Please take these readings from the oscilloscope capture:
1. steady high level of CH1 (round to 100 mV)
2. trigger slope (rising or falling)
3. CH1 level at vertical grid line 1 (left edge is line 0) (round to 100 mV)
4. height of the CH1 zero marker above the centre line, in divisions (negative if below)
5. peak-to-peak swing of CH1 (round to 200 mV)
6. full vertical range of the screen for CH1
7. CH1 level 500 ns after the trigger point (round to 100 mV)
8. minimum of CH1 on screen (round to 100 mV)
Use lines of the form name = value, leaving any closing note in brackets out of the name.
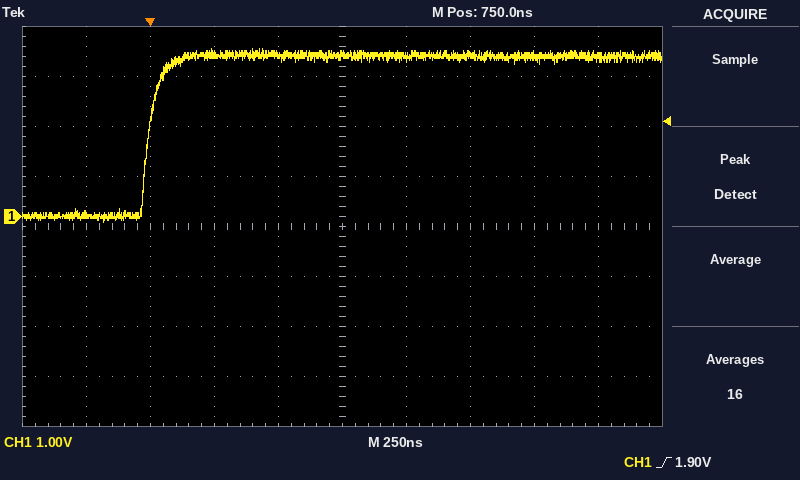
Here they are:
steady high level of CH1 = 3.2 V
trigger slope = rising
CH1 level at vertical grid line 1 (left edge is line 0) = 0.0 V
height of the CH1 zero marker above the centre line, in divisions = +0.2 div
peak-to-peak swing of CH1 = 3.4 V
full vertical range of the screen for CH1 = 8 V
CH1 level 500 ns after the trigger point = 3.2 V
minimum of CH1 on screen = -100 mV
